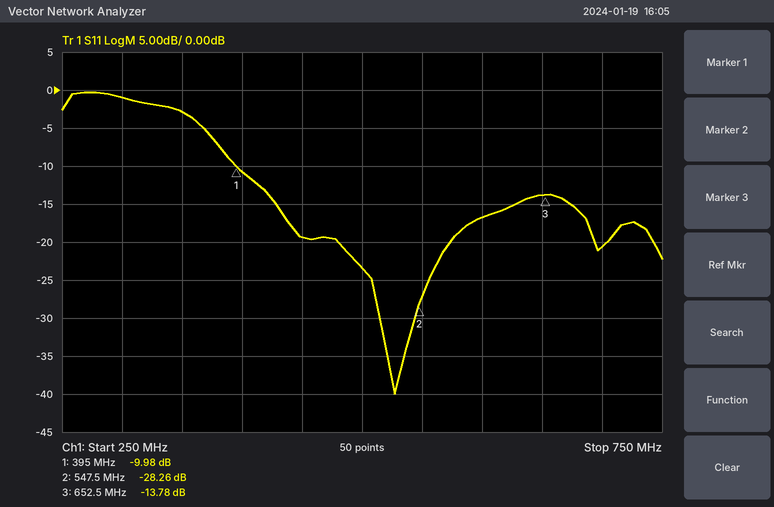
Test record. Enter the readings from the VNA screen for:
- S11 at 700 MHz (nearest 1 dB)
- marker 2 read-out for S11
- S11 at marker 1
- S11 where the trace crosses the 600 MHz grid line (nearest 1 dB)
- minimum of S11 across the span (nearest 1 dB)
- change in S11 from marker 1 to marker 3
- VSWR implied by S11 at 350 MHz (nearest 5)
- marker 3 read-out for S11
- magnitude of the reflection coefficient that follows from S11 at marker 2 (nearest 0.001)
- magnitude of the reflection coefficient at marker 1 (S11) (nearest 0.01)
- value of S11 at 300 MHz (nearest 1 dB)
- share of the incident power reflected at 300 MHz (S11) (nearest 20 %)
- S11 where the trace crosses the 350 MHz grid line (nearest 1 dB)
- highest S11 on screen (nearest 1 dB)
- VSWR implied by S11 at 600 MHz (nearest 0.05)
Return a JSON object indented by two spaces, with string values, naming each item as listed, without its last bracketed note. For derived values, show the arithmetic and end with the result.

{
  "S11 at 700 MHz": "-21 dB",
  "marker 2 read-out for S11": "-28.26 dB",
  "S11 at marker 1": "-9.98 dB",
  "S11 where the trace crosses the 600 MHz grid line": "-17 dB",
  "minimum of S11 across the span": "-40 dB",
  "change in S11 from marker 1 to marker 3": "-13.78 − (-9.98) = -3.80 dB",
  "VSWR implied by S11 at 350 MHz": "|Γ| = 10^(-3/20) = 0.7079; VSWR = (1 + 0.7079)/(1 − 0.7079) ≈ 5.85, so 5 to the nearest 5",
  "marker 3 read-out for S11": "-13.78 dB",
  "magnitude of the reflection coefficient that follows from S11 at marker 2": "10^(-28.26/20) ≈ 0.039",
  "magnitude of the reflection coefficient at marker 1 (S11)": "10^(-9.98/20) ≈ 0.32",
  "value of S11 at 300 MHz": "-1 dB",
  "share of the incident power reflected at 300 MHz (S11)": "10^(-1/10) ≈ 79.4 %, so 80 % to the nearest 20 %",
  "S11 where the trace crosses the 350 MHz grid line": "-3 dB",
  "highest S11 on screen": "0 dB",
  "VSWR implied by S11 at 600 MHz": "|Γ| = 10^(-17/20) = 0.1413; VSWR = (1 + 0.1413)/(1 − 0.1413) ≈ 1.33, so 1.35 to the nearest 0.05"
}
